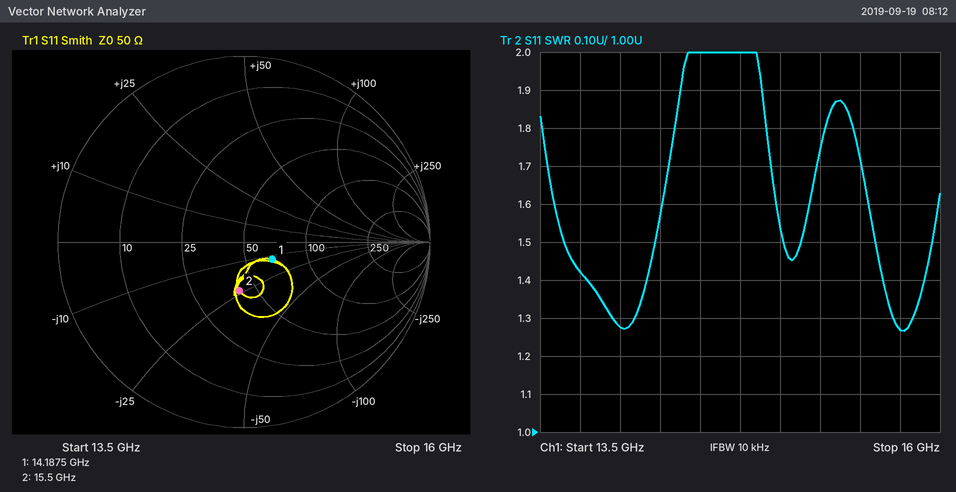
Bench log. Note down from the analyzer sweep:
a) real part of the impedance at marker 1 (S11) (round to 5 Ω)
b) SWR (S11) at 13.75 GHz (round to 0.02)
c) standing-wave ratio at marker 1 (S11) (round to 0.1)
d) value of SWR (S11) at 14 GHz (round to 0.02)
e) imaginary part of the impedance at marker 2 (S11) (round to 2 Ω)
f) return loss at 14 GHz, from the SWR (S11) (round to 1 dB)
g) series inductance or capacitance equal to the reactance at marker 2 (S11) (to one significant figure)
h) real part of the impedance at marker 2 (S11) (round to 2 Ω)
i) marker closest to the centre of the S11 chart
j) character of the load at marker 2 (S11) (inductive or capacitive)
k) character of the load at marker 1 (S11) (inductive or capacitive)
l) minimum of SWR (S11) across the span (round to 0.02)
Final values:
65 Ω
1.42
1.4
1.28
-24 Ω
18 dB
400 fF
42 Ω
marker 1
capacitive
capacitive
1.26
